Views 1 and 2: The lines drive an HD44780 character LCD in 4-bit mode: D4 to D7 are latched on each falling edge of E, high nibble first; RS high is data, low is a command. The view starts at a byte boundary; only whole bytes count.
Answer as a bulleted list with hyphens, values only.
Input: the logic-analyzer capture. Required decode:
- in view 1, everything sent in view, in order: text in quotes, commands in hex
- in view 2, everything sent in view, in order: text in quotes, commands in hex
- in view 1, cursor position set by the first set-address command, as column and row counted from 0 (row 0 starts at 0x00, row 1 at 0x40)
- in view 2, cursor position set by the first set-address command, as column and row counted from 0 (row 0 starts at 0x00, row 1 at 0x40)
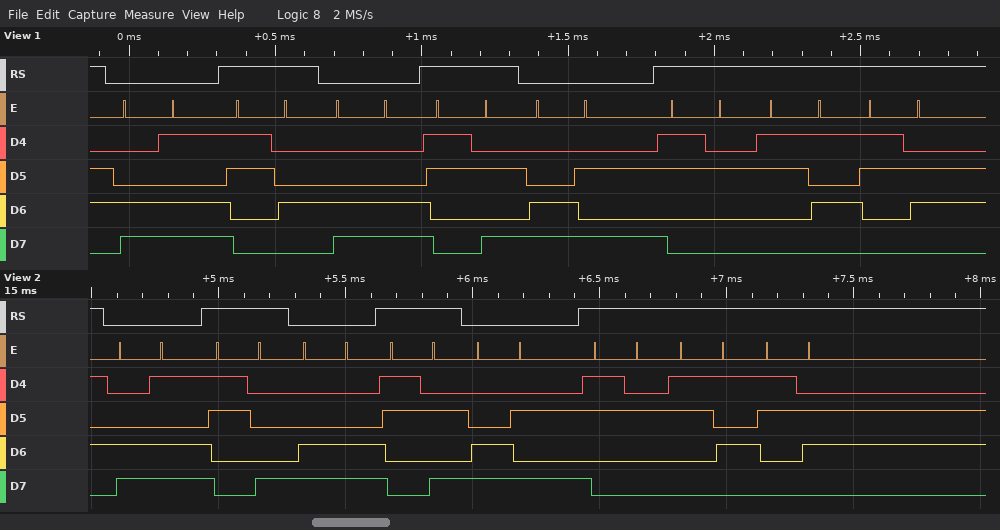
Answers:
- 0xCD "4" 0xCC ":" 0xCA "256"
- 0xCD "8" 0xCC ":" 0xCA "256"
- column 13, row 1
- column 13, row 1
